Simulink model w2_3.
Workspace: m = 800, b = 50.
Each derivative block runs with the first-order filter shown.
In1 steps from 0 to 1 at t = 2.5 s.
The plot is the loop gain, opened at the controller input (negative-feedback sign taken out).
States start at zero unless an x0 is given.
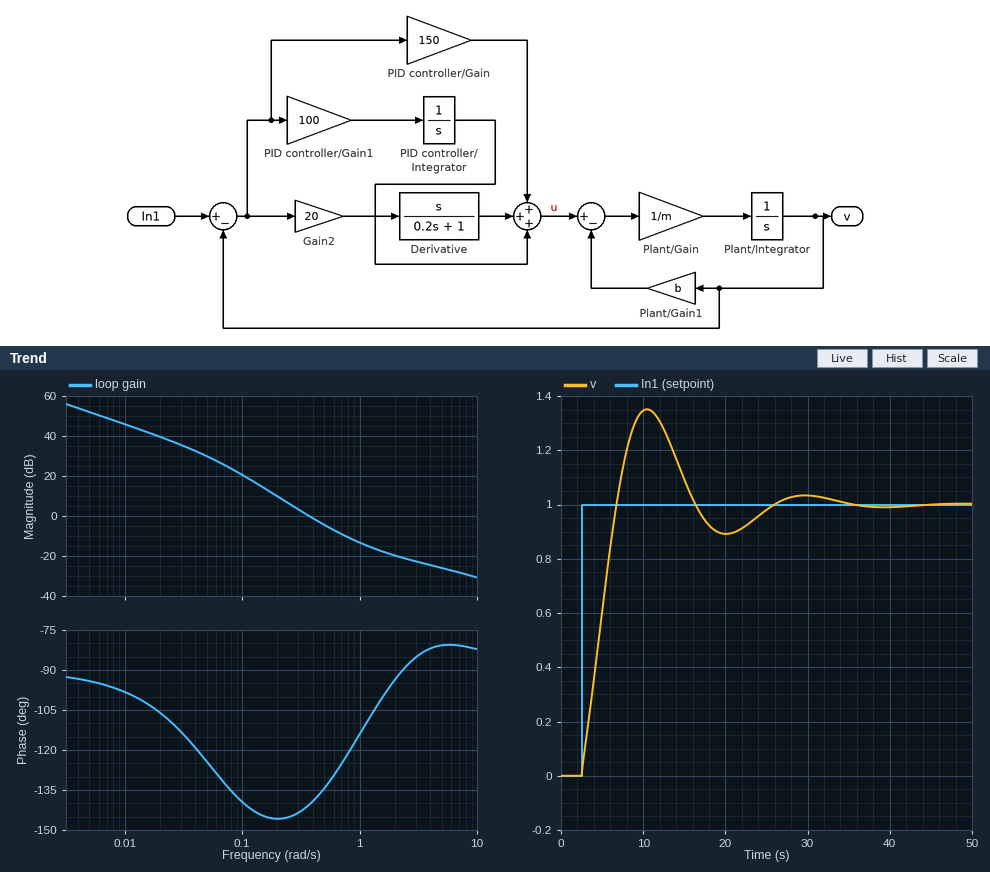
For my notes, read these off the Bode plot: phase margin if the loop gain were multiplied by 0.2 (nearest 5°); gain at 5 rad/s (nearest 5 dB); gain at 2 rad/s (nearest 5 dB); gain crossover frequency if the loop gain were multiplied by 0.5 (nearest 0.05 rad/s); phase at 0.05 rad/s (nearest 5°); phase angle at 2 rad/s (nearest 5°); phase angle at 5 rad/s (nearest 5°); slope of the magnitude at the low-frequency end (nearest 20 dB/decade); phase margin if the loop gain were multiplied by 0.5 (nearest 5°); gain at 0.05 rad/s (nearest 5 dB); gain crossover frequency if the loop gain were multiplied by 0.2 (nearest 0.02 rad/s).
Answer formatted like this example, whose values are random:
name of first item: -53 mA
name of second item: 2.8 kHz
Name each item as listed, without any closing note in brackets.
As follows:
phase margin if the loop gain were multiplied by 0.2: 35°
gain at 5 rad/s: -25 dB
gain at 2 rad/s: -20 dB
gain crossover frequency if the loop gain were multiplied by 0.5: 0.25 rad/s
phase at 0.05 rad/s: -125°
phase angle at 2 rad/s: -95°
phase angle at 5 rad/s: -80°
slope of the magnitude at the low-frequency end: -20 dB/decade
phase margin if the loop gain were multiplied by 0.5: 35°
gain at 0.05 rad/s: 30 dB
gain crossover frequency if the loop gain were multiplied by 0.2: 0.16 rad/s
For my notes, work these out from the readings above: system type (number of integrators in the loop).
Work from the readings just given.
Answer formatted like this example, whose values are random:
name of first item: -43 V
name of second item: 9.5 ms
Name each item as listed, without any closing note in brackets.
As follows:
system type: 1
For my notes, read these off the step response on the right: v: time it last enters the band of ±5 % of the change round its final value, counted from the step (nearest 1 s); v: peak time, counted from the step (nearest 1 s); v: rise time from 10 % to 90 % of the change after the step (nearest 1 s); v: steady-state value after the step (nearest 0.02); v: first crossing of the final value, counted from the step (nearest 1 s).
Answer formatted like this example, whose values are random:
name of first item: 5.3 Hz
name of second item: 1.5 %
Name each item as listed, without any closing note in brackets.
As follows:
v: time it last enters the band of ±5 % of the change round its final value, counted from the step: 21 s
v: peak time, counted from the step: 8 s
v: rise time from 10 % to 90 % of the change after the step: 3 s
v: steady-state value after the step: 1.00
v: first crossing of the final value, counted from the step: 4 s
